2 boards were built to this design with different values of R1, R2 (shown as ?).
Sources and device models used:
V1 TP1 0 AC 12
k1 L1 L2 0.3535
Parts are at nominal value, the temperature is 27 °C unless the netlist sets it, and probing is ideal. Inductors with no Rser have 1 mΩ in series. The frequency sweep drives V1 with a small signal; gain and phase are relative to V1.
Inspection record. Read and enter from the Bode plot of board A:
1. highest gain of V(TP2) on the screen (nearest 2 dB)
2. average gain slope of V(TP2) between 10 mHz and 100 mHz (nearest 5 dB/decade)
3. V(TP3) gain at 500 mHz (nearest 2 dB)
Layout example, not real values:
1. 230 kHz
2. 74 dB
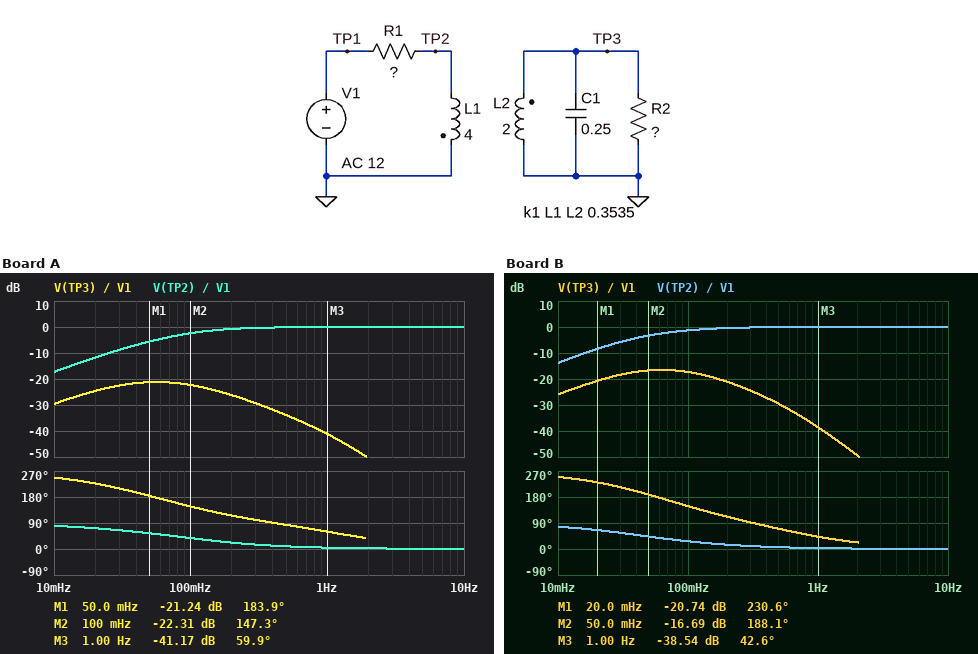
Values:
1. 0 dB
2. 15 dB/decade
3. -34 dB
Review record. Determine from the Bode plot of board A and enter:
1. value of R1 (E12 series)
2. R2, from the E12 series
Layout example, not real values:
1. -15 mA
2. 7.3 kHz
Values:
1. 1.8 Ω
2. 0.47 Ω
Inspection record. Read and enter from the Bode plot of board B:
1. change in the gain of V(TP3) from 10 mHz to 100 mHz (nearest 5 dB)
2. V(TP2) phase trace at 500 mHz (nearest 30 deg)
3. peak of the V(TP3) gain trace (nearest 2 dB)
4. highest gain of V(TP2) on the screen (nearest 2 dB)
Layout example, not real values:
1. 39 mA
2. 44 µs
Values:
1. 10 dB
2. 0 deg
3. -16 dB
4. 0 dB
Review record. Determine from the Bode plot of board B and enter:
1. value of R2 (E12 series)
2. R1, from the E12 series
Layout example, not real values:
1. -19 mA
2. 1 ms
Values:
1. 0.82 Ω
2. 1.2 Ω
